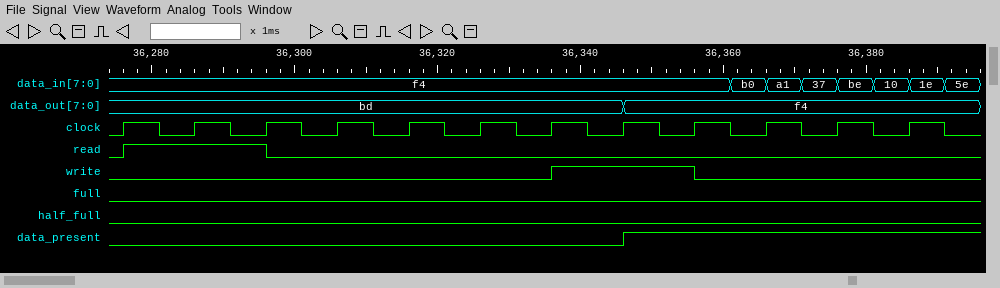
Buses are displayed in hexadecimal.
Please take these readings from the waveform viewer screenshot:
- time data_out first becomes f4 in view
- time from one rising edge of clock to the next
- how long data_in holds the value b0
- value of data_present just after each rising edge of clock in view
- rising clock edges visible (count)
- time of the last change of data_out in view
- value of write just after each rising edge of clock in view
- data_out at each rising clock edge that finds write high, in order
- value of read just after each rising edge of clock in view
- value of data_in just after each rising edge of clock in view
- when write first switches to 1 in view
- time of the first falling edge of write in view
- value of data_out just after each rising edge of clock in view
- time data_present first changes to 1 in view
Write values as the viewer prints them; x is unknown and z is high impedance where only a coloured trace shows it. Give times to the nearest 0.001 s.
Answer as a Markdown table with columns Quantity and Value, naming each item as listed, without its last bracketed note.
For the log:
| Quantity | Value |
|---|---|
| time data_out first becomes f4 in view | 36.346 s |
| time from one rising edge of clock to the next | 0.01 s |
| how long data_in holds the value b0 | 0.005 s |
| value of data_present just after each rising edge of clock in view | 0 0 0 0 0 0 0 1 1 1 1 1 |
| rising clock edges visible | 12 |
| time of the last change of data_out in view | 36.346 s |
| value of write just after each rising edge of clock in view | 0 0 0 0 0 0 1 1 0 0 0 0 |
| data_out at each rising clock edge that finds write high, in order | bd, f4 |
| value of read just after each rising edge of clock in view | 1 1 0 0 0 0 0 0 0 0 0 0 |
| value of data_in just after each rising edge of clock in view | f4, f4, f4, f4, f4, f4, f4, f4, f4, a1, be, 1e |
| when write first switches to 1 in view | 36.336 s |
| time of the first falling edge of write in view | 36.356 s |
| value of data_out just after each rising edge of clock in view | bd, bd, bd, bd, bd, bd, bd, f4, f4, f4, f4, f4 |
| time data_present first changes to 1 in view | 36.346 s |
